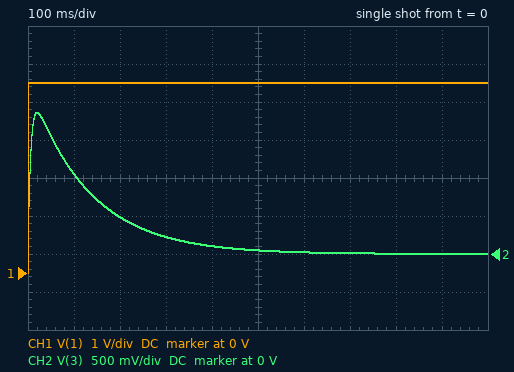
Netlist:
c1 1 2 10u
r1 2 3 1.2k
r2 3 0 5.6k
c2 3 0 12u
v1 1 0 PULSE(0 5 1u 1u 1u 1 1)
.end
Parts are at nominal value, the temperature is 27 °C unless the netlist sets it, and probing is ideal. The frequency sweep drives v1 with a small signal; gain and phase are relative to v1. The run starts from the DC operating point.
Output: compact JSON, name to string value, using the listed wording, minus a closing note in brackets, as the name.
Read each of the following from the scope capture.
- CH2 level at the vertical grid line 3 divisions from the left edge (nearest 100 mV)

{"CH2 level at the vertical grid line 3 divisions from the left edge": "200 mV"}
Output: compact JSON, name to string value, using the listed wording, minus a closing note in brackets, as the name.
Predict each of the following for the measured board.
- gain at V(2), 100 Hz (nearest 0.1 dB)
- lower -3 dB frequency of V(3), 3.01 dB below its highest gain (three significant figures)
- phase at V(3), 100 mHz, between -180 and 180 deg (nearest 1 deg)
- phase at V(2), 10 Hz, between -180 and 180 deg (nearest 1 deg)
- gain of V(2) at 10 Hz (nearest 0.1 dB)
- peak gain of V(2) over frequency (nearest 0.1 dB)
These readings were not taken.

{"gain at V(2), 100 Hz": "-0.2 dB", "lower -3 dB frequency of V(3), 3.01 dB below its highest gain": "1.13 Hz", "phase at V(3), 100 mHz, between -180 and 180 deg": "85 deg", "phase at V(2), 10 Hz, between -180 and 180 deg": "22 deg", "gain of V(2) at 10 Hz": "-4.3 dB", "peak gain of V(2) over frequency": "0 dB"}
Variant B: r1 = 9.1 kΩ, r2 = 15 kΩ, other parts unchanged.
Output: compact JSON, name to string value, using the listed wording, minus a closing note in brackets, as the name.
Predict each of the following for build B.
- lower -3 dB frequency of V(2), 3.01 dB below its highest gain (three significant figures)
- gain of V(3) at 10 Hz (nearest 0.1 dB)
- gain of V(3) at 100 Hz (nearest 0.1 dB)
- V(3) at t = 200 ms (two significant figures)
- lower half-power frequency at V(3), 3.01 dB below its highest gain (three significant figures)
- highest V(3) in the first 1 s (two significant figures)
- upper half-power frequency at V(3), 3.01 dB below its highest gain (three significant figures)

{"lower -3 dB frequency of V(2), 3.01 dB below its highest gain": "1.84 Hz", "gain of V(3) at 10 Hz": "-17.3 dB", "gain of V(3) at 100 Hz": "-36.7 dB", "V(3) at t = 200 ms": "1.3 V", "lower half-power frequency at V(3), 3.01 dB below its highest gain": "348 mHz", "highest V(3) in the first 1 s": "1.5 V", "upper half-power frequency at V(3), 3.01 dB below its highest gain": "4.44 Hz"}
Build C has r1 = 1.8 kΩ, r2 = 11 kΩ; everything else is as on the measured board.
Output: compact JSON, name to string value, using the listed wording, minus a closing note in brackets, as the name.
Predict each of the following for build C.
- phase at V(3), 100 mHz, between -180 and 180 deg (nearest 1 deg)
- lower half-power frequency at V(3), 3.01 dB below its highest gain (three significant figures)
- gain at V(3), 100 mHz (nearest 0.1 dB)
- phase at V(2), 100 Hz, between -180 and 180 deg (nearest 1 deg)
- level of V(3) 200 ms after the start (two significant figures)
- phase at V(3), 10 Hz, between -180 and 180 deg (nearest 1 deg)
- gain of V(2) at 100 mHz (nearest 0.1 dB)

{"phase at V(3), 100 mHz, between -180 and 180 deg": "81 deg", "lower half-power frequency at V(3), 3.01 dB below its highest gain": "592 mHz", "gain at V(3), 100 mHz": "-23.3 dB", "phase at V(2), 100 Hz, between -180 and 180 deg": "5 deg", "level of V(3) 200 ms after the start": "1.0 V", "phase at V(3), 10 Hz, between -180 and 180 deg": "-27 deg", "gain of V(2) at 100 mHz": "-22.0 dB"}
